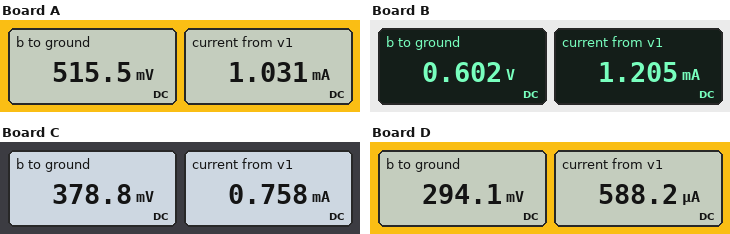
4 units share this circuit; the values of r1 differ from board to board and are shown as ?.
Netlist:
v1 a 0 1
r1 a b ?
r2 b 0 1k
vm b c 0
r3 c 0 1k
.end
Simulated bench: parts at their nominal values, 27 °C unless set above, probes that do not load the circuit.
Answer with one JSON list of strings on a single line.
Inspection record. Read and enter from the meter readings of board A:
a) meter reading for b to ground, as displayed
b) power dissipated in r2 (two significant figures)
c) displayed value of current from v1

["515.5 mV", "270 µW", "1.031 mA"]
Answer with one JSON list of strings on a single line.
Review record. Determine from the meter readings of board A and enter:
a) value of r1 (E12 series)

["470 Ω"]
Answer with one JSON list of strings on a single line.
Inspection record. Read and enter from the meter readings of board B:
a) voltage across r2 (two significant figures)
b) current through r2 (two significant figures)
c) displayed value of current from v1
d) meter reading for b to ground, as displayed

["600 mV", "600 µA", "1.205 mA", "0.602 V"]
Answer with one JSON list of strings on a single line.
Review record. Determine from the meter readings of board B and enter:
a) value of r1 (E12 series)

["330 Ω"]
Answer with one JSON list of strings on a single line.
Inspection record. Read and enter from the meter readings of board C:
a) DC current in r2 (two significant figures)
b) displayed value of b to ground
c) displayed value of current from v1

["380 µA", "378.8 mV", "0.758 mA"]
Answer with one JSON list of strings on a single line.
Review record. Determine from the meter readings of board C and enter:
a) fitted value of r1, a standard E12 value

["820 Ω"]
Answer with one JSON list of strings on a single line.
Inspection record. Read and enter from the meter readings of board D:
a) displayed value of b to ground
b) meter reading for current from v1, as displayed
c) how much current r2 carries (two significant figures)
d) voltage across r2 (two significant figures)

["294.1 mV", "588.2 µA", "290 µA", "290 mV"]
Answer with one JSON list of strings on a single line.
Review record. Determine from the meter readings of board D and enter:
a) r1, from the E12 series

["1.2 kΩ"]
